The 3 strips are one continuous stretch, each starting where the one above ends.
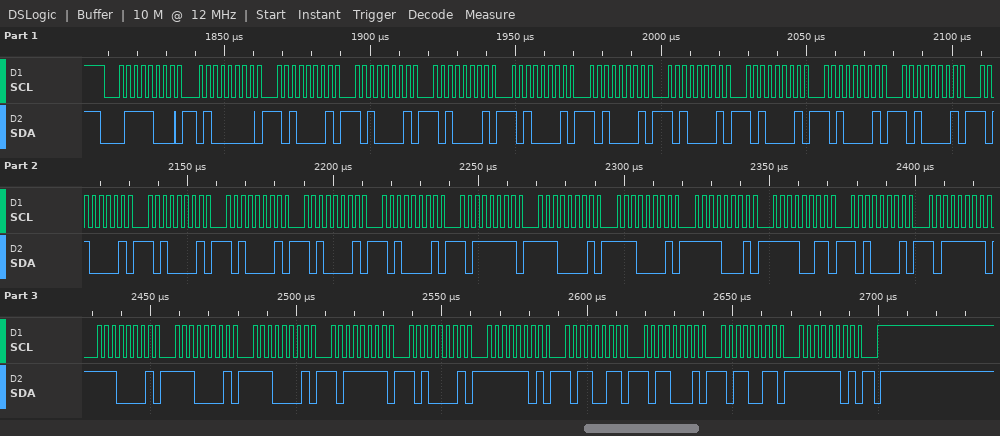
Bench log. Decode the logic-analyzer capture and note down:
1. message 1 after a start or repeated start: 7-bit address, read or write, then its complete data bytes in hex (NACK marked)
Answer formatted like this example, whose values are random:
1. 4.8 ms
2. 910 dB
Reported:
1. 0x3C write: 40 A1 A1 A1 A1 A1 A1 A1 A1 A1 A1 A1 A1 A1 A1 BF E1 E1 F1 F3 A1 BF E1 E1 E1 BF A1 FD B3 B1 B3 FD
